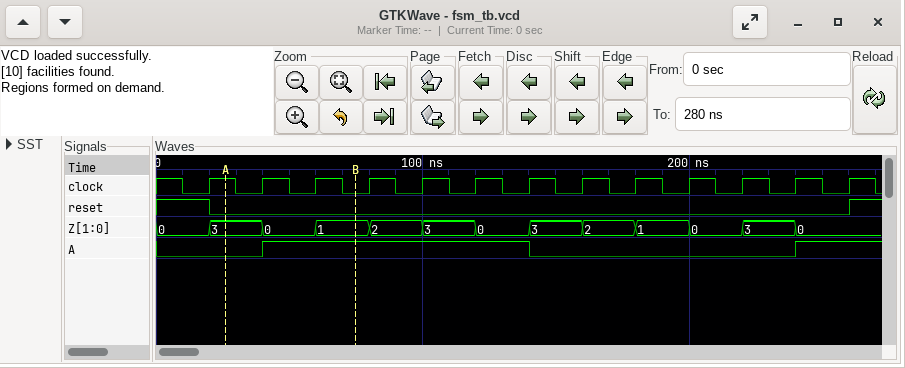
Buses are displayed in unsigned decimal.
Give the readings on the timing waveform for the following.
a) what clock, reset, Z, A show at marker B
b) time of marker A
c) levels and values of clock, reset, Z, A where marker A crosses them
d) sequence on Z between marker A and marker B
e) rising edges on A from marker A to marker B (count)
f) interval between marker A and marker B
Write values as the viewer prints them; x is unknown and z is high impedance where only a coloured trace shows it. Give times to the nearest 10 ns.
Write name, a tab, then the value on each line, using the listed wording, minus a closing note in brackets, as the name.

what clock, reset, Z, A show at marker B	clock=0, reset=0, Z=1, A=1
time of marker A	30 ns
levels and values of clock, reset, Z, A where marker A crosses them	clock=1, reset=0, Z=3, A=0
sequence on Z between marker A and marker B	3, 0, 1
rising edges on A from marker A to marker B	1
interval between marker A and marker B	50 ns
